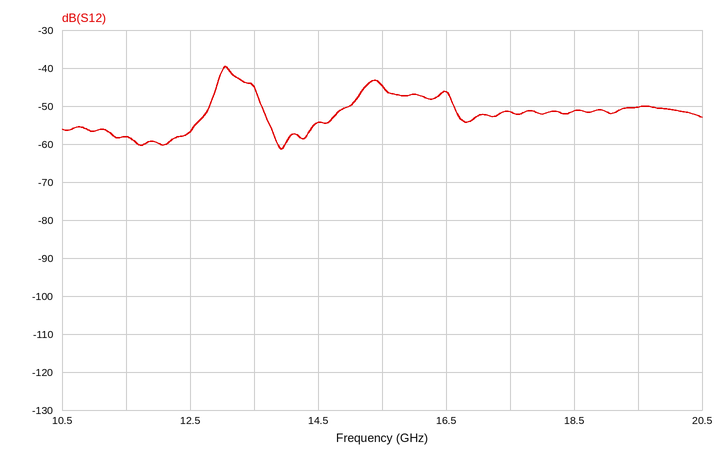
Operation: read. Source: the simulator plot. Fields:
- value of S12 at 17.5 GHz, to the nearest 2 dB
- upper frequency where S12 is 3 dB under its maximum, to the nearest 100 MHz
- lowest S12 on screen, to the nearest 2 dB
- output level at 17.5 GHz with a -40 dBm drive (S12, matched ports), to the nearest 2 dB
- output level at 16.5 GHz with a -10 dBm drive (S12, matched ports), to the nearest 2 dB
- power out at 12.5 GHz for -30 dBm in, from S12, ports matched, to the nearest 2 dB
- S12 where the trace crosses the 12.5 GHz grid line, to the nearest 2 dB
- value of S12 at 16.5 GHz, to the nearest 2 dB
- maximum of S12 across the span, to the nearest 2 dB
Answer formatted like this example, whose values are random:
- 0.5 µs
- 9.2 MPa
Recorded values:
- -52 dB
- 13.2 GHz
- -62 dB
- -92 dBm
- -56 dBm
- -86 dBm
- -56 dB
- -46 dB
- -40 dB
